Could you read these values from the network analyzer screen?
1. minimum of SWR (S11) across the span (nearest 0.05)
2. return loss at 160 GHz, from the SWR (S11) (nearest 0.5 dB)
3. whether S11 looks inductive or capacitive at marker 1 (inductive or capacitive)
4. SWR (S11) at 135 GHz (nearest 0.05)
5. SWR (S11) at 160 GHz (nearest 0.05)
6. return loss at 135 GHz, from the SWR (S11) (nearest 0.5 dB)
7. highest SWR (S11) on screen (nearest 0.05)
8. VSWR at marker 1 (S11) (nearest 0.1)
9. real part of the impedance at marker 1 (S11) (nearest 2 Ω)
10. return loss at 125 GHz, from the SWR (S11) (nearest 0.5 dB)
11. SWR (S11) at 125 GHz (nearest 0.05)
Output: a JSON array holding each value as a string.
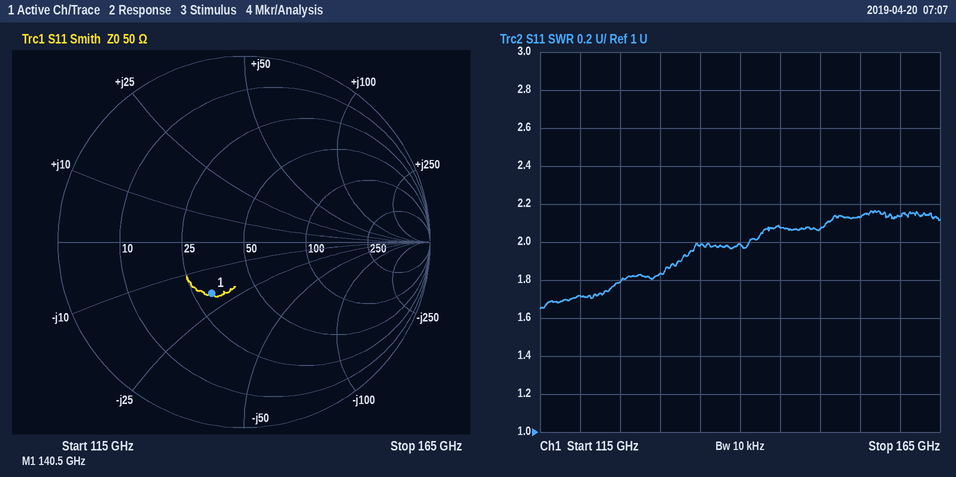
["1.65", "9.0 dB", "capacitive", "2.00", "2.15", "9.5 dB", "2.15", "2.0", "30 Ω", "11.0 dB", "1.80"]
